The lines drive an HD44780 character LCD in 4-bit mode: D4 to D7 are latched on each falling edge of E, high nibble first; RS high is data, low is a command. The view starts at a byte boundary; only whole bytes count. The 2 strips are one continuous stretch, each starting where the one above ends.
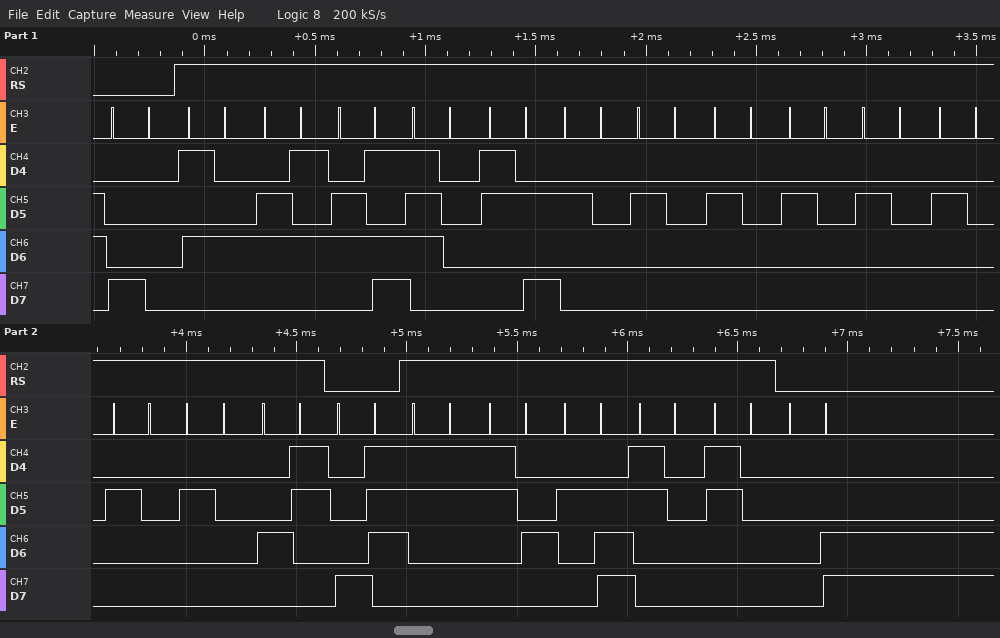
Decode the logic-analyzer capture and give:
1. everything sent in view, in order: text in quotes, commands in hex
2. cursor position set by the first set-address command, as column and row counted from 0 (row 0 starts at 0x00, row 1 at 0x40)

0x80 "Temp:        C" 0x87 "34.00" 0x0C
column 0, row 0
